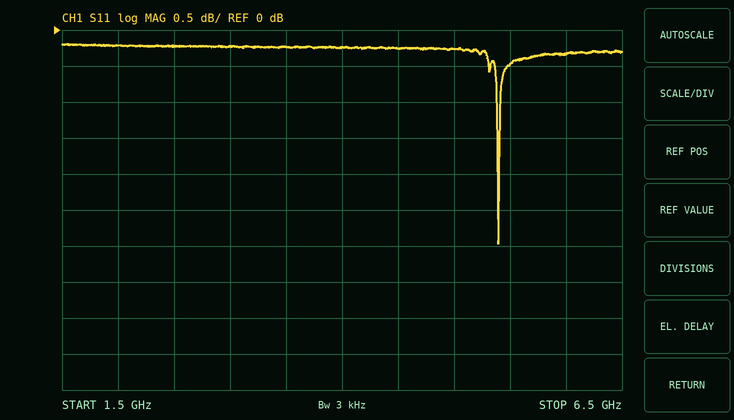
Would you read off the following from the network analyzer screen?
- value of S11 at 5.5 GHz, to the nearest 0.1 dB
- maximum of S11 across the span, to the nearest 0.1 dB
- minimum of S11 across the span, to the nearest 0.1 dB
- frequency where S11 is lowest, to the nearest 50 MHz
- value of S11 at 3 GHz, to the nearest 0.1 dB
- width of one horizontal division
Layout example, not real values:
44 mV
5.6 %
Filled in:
-0.5 dB
-0.2 dB
-3.0 dB
5.40 GHz
-0.2 dB
500 MHz
